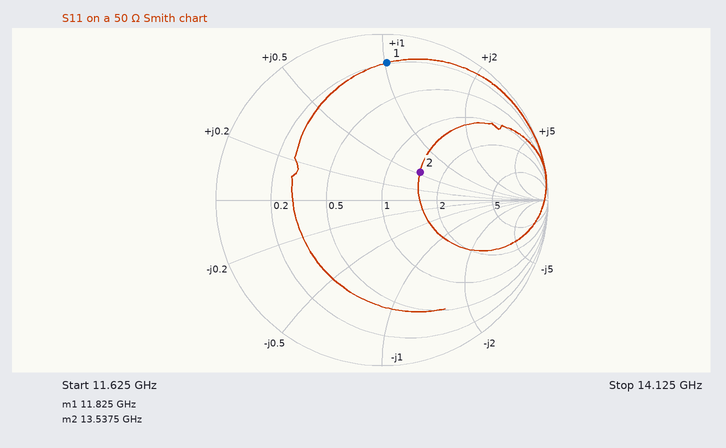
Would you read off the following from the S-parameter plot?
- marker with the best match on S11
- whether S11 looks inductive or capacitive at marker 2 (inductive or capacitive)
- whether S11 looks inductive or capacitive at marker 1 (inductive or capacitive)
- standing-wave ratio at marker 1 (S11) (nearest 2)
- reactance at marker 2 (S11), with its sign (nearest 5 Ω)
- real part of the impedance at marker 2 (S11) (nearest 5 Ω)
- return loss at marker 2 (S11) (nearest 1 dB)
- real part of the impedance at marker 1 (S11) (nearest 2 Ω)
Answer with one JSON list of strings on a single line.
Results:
["marker 2", "inductive", "inductive", "10", "+25 Ω", "75 Ω", "11 dB", "10 Ω"]
